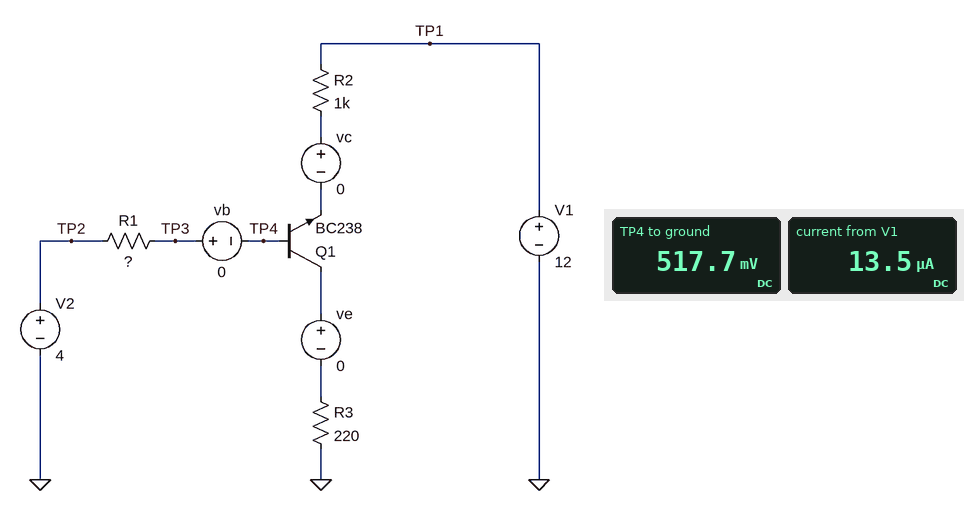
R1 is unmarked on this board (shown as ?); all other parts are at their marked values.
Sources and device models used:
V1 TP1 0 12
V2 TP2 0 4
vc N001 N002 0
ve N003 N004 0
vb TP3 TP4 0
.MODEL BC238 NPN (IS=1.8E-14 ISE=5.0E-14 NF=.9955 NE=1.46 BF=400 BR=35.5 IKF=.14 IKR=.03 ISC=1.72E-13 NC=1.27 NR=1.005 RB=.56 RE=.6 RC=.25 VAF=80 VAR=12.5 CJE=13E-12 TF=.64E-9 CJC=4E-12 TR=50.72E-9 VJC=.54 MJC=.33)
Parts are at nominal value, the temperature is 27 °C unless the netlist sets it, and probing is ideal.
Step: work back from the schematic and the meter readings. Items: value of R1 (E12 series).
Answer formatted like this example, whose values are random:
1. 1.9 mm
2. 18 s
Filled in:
1. 2.7 MΩ
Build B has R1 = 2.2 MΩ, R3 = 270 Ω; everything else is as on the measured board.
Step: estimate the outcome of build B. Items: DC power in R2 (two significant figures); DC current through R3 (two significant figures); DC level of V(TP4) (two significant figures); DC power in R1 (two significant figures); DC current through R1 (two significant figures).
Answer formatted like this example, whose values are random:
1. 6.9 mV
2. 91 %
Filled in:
1. 300 nW
2. 19 µA
3. 530 mV
4. 5.5 µW
5. 1.6 µA
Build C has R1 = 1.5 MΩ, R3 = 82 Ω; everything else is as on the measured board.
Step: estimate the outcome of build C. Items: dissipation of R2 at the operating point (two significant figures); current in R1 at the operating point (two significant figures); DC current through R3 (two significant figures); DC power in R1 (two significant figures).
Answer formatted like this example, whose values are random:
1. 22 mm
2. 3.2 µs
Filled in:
1. 750 nW
2. 2.3 µA
3. 30 µA
4. 8.0 µW
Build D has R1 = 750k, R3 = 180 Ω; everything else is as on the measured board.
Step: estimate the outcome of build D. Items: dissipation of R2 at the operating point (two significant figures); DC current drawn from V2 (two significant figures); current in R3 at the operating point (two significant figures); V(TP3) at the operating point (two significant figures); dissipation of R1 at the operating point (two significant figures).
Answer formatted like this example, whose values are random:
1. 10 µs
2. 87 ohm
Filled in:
1. 3.9 µW
2. 4.6 µA
3. 67 µA
4. 570 mV
5. 16 µW
